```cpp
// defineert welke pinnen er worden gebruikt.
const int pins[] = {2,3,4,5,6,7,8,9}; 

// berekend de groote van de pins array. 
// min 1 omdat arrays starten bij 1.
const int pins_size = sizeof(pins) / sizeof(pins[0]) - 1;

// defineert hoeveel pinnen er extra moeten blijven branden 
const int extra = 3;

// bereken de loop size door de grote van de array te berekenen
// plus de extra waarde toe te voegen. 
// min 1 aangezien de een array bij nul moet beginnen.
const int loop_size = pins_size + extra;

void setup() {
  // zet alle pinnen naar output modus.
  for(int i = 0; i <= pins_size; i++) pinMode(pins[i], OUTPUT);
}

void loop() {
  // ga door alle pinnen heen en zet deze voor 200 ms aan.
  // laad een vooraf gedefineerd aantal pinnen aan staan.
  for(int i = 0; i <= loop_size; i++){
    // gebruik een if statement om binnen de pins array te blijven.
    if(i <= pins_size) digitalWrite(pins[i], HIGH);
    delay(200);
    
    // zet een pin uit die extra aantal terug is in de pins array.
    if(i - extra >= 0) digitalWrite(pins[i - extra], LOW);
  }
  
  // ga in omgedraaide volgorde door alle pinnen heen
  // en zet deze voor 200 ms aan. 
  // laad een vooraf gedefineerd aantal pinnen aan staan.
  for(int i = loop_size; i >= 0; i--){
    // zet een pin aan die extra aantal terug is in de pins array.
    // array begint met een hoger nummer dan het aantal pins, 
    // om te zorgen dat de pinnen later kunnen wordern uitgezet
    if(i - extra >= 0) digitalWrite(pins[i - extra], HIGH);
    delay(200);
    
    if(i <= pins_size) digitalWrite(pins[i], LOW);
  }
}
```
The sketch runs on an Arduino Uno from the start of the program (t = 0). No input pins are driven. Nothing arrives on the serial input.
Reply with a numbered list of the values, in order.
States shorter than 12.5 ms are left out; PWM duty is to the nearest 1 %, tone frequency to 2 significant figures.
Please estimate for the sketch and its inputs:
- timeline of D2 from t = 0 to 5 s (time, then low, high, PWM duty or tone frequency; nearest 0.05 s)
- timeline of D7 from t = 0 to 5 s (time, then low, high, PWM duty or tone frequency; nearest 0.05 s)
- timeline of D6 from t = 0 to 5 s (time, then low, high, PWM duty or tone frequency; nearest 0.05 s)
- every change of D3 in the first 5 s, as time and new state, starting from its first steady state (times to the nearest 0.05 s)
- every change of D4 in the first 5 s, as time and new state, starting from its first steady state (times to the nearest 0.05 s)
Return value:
1. 0 s high; 0.8 s low; 3.6 s high
2. 0 s low; 1 s high; 1.8 s low; 2.6 s high; 3.4 s low
3. 0 s low; 0.8 s high; 1.6 s low; 2.8 s high; 3.6 s low
4. 0 s low; 0.2 s high; 1 s low; 3.4 s high; 4.2 s low; 4.6 s high
5. 0 s low; 0.4 s high; 1.2 s low; 3.2 s high; 4 s low; 4.8 s high
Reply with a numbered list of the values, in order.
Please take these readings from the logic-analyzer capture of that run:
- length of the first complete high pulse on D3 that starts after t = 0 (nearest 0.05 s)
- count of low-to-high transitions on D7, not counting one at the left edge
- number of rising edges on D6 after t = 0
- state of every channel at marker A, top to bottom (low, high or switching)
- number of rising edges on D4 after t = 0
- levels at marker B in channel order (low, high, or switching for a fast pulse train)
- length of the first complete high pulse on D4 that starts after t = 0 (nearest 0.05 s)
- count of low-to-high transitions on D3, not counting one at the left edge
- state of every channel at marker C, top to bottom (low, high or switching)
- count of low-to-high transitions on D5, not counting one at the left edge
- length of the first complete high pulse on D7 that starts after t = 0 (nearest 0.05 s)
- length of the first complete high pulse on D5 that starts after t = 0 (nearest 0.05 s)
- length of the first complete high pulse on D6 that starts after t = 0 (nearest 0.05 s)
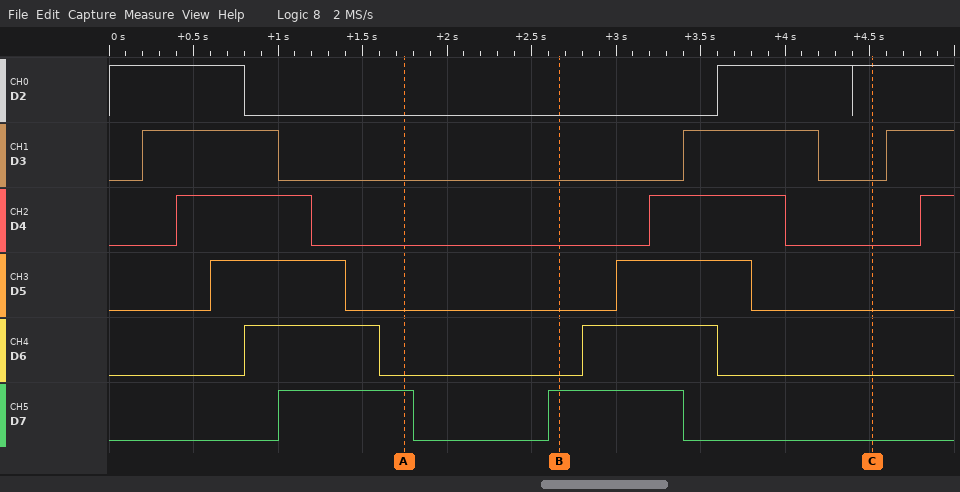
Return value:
1. 0.80 s
2. 2
3. 2
4. D2 low, D3 low, D4 low, D5 low, D6 low, D7 high
5. 3
6. D2 low, D3 low, D4 low, D5 low, D6 low, D7 high
7. 0.80 s
8. 3
9. D2 high, D3 low, D4 low, D5 low, D6 low, D7 low
10. 2
11. 0.80 s
12. 0.80 s
13. 0.80 s
